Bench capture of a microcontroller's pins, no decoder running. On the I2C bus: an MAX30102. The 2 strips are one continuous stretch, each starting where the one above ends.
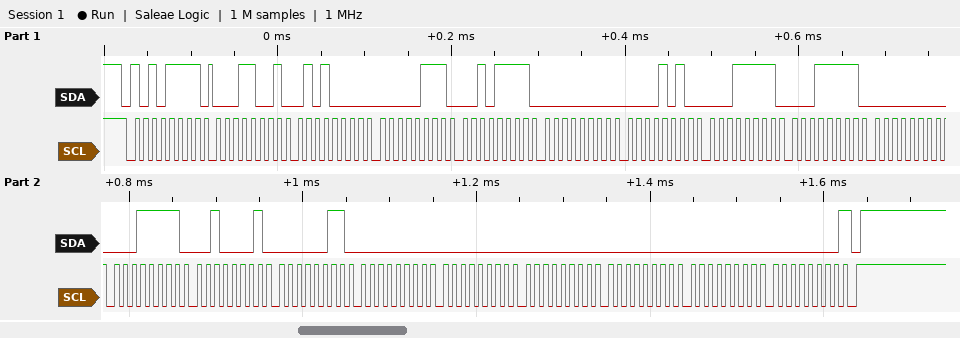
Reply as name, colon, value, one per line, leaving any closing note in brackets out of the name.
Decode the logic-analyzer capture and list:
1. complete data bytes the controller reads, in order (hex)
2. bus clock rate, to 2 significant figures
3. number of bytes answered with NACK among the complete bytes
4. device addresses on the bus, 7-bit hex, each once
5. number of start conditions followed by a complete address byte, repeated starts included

complete data bytes the controller reads, in order: 19 50 07 2F 00 0A 1F 1F 00 1F 21 03 00 00 00 00 00 00
bus clock rate, to 2 significant figures: 100 kHz
number of bytes answered with NACK among the complete bytes: 1
device addresses on the bus, 7-bit hex, each once: 0x57
number of start conditions followed by a complete address byte, repeated starts included: 1
